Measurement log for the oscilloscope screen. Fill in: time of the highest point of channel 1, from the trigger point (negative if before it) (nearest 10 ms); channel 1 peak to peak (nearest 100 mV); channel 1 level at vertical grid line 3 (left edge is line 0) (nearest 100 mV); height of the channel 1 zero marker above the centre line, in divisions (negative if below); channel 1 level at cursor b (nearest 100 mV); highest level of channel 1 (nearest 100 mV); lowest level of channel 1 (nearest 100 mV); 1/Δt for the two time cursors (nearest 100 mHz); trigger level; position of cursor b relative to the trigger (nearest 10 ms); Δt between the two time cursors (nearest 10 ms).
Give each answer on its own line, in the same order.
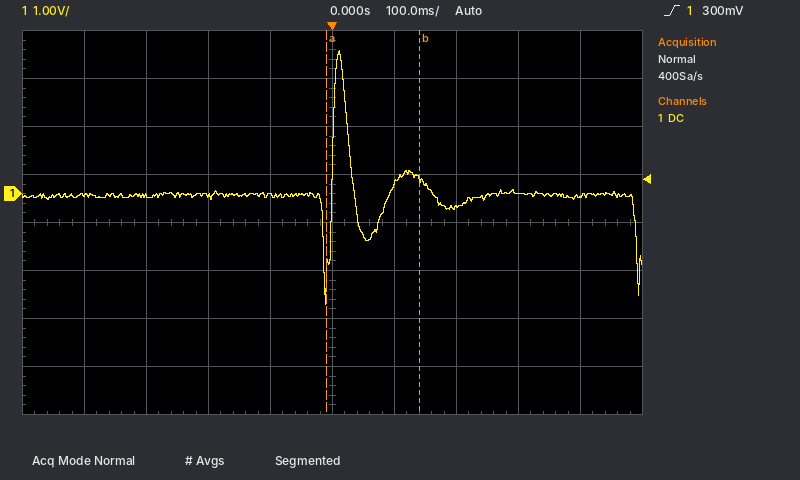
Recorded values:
+10 ms
5.3 V
-100 mV
+0.6 div
300 mV
3.0 V
-2.3 V
6.7 Hz
300 mV
+140 ms
150 ms
